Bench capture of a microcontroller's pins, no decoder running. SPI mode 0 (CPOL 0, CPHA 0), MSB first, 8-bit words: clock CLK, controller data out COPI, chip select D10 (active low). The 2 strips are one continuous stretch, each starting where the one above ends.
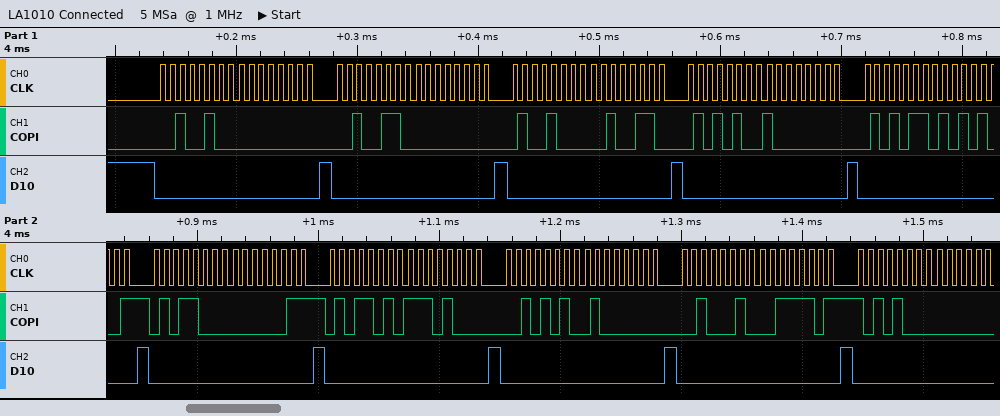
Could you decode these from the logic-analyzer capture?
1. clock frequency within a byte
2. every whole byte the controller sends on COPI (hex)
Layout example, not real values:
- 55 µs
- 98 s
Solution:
- 125 kHz
- 24 00 26 00 48 26 54 80 56 A9 58 03 5A E8 2A 40 22 3D A8
